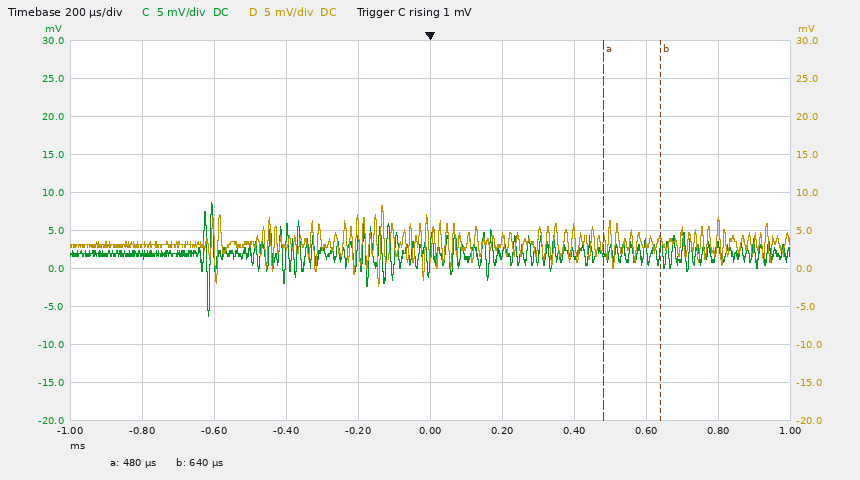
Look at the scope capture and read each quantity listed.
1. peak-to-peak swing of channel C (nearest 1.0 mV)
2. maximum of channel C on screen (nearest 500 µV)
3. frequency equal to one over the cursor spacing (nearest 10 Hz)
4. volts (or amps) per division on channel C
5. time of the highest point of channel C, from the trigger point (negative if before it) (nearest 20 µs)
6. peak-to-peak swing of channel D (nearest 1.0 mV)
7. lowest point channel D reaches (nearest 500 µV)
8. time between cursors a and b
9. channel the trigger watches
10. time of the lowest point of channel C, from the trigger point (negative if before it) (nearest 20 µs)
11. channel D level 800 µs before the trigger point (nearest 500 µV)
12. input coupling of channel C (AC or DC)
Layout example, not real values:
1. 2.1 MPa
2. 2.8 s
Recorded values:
1. 15.0 mV
2. 8.5 mV
3. 6.25 kHz
4. 5 mV
5. -600 µs
6. 11.0 mV
7. -2.5 mV
8. 160 µs
9. channel C
10. -620 µs
11. 3.0 mV
12. DC
